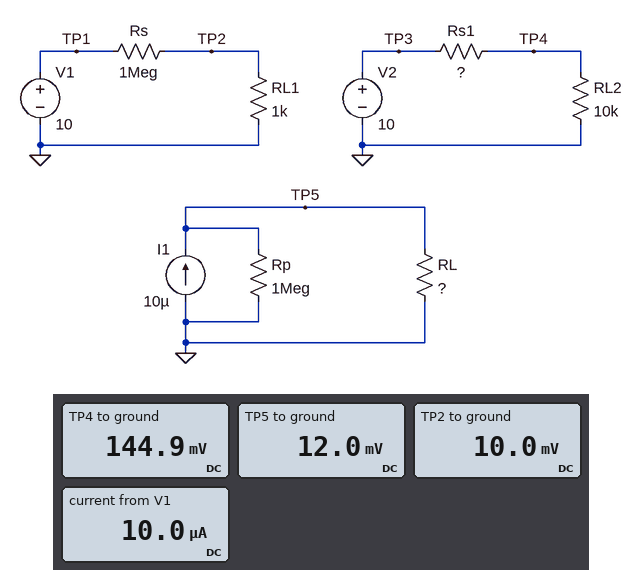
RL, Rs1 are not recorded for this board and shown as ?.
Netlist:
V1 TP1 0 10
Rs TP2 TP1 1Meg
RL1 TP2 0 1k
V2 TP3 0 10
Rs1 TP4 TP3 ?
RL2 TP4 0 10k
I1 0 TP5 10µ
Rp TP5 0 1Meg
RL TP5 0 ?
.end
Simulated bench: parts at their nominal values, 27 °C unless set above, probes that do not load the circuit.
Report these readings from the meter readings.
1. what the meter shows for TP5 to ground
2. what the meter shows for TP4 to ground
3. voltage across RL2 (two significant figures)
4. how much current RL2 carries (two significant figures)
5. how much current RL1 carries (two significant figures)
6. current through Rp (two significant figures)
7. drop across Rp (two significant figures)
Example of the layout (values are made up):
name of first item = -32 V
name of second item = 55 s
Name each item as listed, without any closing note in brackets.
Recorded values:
what the meter shows for TP5 to ground = 12.0 mV
what the meter shows for TP4 to ground = 144.9 mV
voltage across RL2 = 140 mV
how much current RL2 carries = 14 µA
how much current RL1 carries = 10 µA
current through Rp = 12 nA
drop across Rp = 12 mV
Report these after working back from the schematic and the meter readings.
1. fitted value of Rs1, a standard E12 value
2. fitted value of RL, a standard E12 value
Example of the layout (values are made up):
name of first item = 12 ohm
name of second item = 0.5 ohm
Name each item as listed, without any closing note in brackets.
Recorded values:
fitted value of Rs1, a standard E12 value = 680 kΩ
fitted value of RL, a standard E12 value = 1.2 kΩ
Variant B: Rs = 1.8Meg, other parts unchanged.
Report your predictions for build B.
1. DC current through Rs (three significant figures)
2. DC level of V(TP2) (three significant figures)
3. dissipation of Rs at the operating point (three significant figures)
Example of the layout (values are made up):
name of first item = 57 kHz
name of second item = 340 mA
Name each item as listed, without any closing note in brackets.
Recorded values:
DC current through Rs = 5.55 µA
DC level of V(TP2) = 5.55 mV
dissipation of Rs at the operating point = 55.5 µW
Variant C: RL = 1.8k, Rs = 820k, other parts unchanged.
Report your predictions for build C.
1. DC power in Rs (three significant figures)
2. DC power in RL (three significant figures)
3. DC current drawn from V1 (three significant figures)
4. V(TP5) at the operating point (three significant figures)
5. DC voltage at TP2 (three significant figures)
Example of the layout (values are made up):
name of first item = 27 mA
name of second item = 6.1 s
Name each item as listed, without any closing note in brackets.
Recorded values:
DC power in Rs = 122 µW
DC power in RL = 179 nW
DC current drawn from V1 = 12.2 µA
V(TP5) at the operating point = 18.0 mV
DC voltage at TP2 = 12.2 mV
